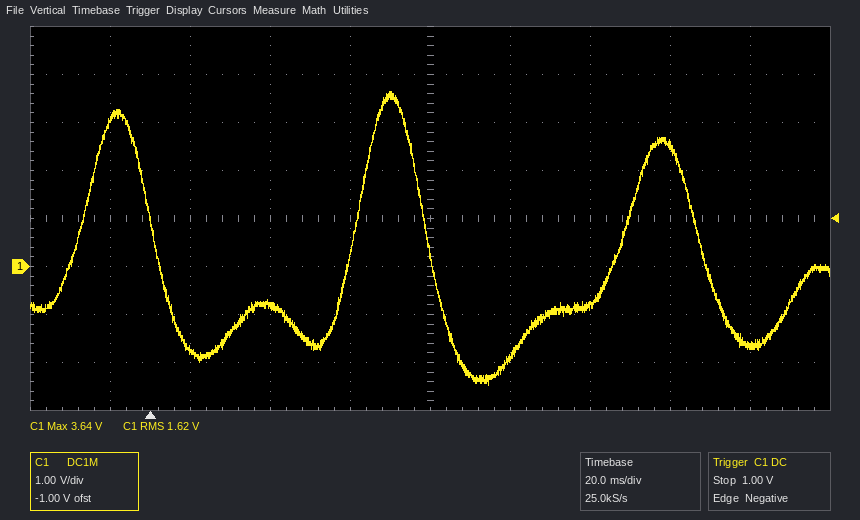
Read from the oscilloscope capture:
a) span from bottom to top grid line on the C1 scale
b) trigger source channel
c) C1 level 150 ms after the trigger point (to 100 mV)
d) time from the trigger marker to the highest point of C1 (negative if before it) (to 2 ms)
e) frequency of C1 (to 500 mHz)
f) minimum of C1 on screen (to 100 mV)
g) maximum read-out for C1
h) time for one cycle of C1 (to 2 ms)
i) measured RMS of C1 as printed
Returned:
8 V
C1
-1.6 V
+60 ms
14.5 Hz
-2.5 V
3.64 V
68 ms
1.62 V
